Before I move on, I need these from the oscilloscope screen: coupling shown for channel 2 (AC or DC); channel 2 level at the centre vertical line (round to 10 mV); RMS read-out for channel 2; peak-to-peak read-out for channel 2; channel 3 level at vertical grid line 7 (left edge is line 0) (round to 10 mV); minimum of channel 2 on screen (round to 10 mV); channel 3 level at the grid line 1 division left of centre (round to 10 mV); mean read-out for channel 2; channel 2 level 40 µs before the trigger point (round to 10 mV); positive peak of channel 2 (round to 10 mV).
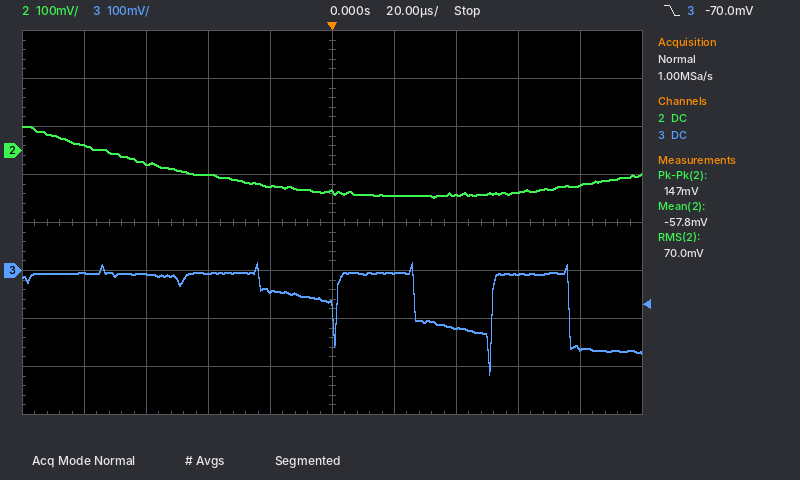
DC
-90 mV
70.0 mV
147 mV
-120 mV
-100 mV
-40 mV
-57.8 mV
-50 mV
50 mV
